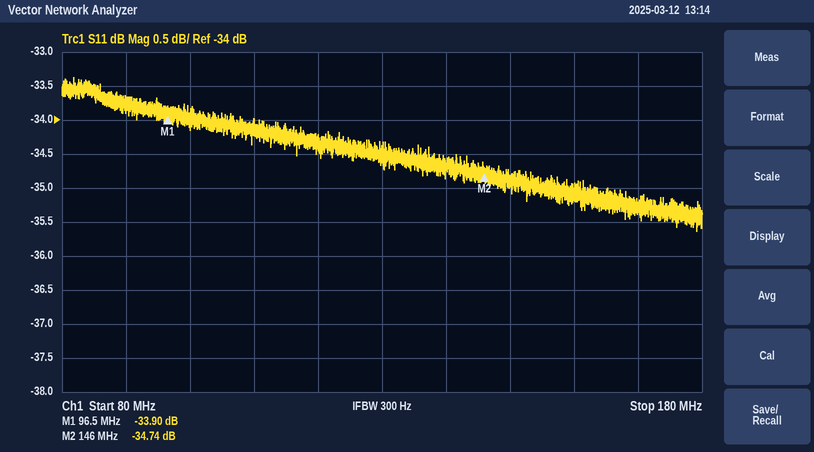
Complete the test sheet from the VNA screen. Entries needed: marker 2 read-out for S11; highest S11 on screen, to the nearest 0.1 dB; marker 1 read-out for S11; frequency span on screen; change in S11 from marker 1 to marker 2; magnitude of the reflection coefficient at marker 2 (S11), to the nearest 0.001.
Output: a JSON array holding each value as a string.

["-34.74 dB", "-33.4 dB", "-33.90 dB", "100 MHz", "-0.84 dB", "0.018"]
